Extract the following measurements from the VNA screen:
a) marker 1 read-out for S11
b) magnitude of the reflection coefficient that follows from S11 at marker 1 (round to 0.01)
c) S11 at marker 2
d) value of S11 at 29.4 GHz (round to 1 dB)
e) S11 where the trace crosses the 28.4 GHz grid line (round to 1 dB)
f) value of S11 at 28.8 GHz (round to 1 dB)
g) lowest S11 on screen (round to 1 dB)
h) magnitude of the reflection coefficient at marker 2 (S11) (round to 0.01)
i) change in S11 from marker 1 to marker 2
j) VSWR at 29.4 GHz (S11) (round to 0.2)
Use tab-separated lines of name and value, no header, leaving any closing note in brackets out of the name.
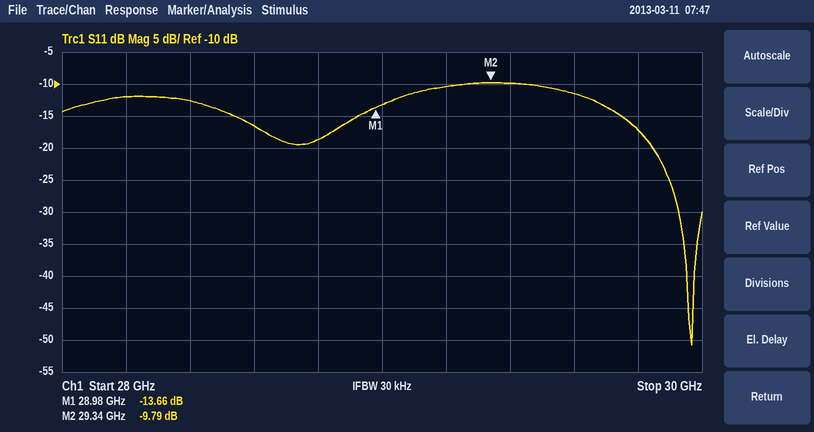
marker 1 read-out for S11	-13.66 dB
magnitude of the reflection coefficient that follows from S11 at marker 1	0.21
S11 at marker 2	-9.79 dB
value of S11 at 29.4 GHz	-10 dB
S11 where the trace crosses the 28.4 GHz grid line	-13 dB
value of S11 at 28.8 GHz	-19 dB
lowest S11 on screen	-51 dB
magnitude of the reflection coefficient at marker 2 (S11)	0.32
change in S11 from marker 1 to marker 2	3.87 dB
VSWR at 29.4 GHz (S11)	2.0
